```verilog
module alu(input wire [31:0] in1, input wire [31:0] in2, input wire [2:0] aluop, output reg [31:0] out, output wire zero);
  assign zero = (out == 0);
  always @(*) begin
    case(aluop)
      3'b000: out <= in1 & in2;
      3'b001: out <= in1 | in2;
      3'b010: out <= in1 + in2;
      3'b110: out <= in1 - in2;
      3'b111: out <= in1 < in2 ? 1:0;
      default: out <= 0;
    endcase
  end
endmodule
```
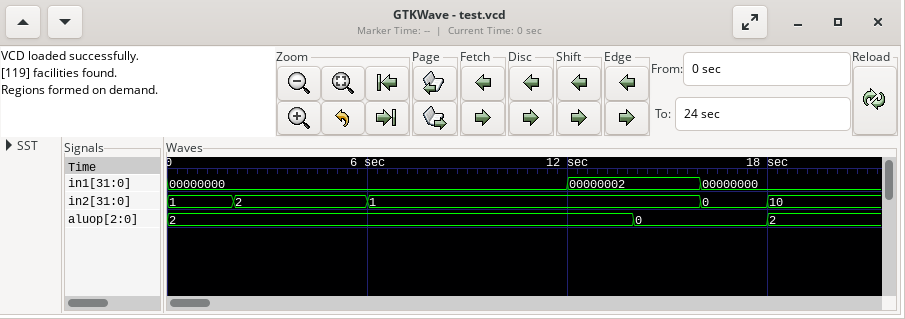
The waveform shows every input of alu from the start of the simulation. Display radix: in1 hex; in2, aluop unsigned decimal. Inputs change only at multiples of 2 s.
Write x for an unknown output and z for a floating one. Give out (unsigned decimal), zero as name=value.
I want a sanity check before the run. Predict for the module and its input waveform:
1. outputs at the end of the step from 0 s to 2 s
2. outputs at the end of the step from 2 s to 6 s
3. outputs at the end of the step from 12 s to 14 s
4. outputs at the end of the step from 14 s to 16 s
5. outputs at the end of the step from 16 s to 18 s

out=1, zero=0
out=2, zero=0
out=3, zero=0
out=0, zero=1
out=0, zero=1
